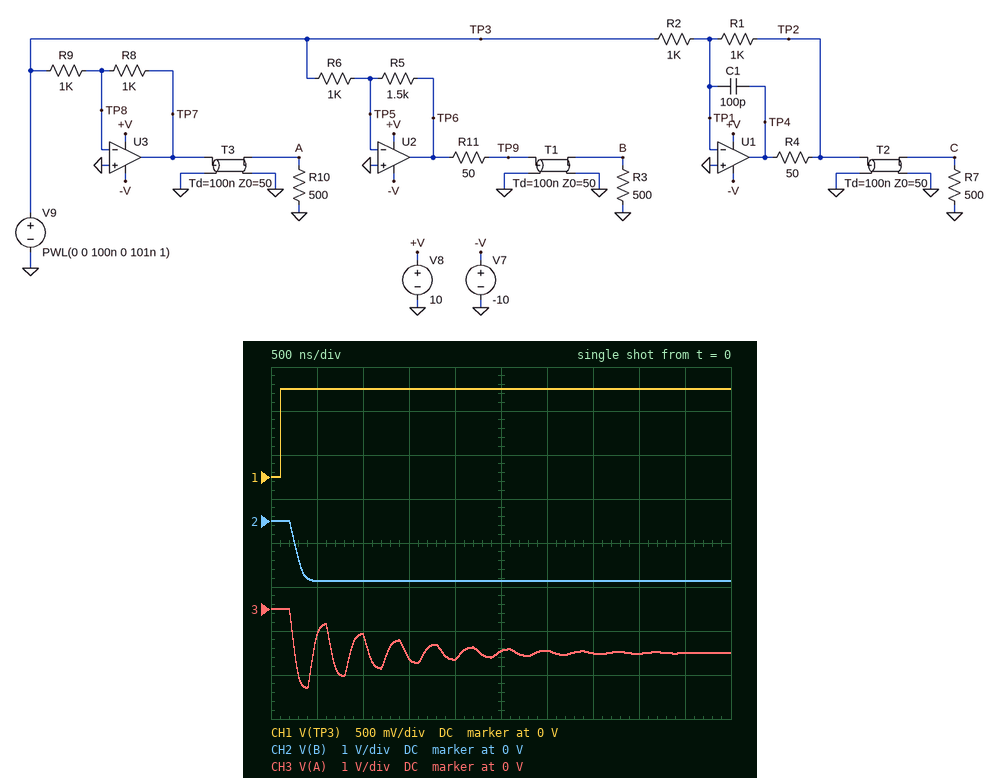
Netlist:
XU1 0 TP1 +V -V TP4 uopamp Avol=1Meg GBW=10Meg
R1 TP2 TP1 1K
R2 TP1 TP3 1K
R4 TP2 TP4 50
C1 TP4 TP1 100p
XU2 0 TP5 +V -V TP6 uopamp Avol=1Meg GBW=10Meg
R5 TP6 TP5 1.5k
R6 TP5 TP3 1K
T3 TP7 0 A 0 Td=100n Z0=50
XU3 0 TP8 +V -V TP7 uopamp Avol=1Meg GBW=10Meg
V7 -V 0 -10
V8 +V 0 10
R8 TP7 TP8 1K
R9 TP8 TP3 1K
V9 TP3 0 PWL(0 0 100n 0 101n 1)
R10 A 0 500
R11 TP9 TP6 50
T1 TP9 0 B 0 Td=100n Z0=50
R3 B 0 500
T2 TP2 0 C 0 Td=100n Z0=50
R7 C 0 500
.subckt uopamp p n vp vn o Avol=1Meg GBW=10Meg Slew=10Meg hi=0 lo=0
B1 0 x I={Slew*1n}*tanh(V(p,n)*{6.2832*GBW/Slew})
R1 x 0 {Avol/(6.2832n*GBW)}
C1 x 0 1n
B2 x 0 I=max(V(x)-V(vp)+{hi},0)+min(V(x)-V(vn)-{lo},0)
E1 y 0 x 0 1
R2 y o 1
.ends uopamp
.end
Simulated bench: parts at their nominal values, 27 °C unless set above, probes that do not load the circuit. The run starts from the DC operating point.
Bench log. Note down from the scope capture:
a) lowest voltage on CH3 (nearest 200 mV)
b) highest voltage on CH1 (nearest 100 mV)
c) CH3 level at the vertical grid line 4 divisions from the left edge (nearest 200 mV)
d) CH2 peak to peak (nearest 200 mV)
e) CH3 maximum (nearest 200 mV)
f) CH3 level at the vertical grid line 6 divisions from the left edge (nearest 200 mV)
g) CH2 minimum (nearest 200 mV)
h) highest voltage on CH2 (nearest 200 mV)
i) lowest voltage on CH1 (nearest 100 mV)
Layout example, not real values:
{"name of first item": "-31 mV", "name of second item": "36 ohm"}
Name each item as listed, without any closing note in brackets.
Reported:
{"lowest voltage on CH3": "-1.8 V", "highest voltage on CH1": "1.0 V", "CH3 level at the vertical grid line 4 divisions from the left edge": "-1.2 V", "CH2 peak to peak": "1.4 V", "CH3 maximum": "0 V", "CH3 level at the vertical grid line 6 divisions from the left edge": "-1.0 V", "CH2 minimum": "-1.4 V", "highest voltage on CH2": "0 V", "lowest voltage on CH1": "0 V"}
